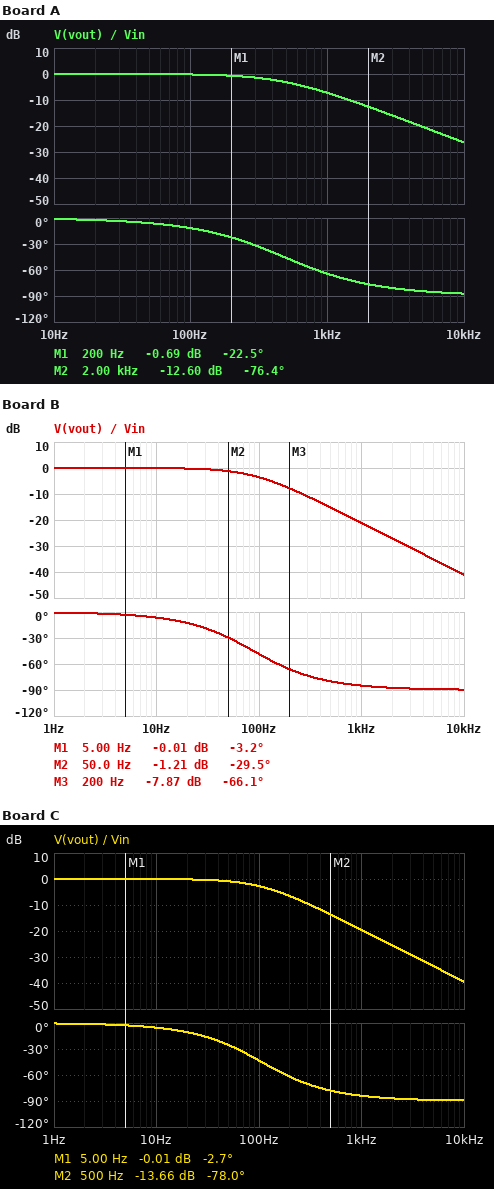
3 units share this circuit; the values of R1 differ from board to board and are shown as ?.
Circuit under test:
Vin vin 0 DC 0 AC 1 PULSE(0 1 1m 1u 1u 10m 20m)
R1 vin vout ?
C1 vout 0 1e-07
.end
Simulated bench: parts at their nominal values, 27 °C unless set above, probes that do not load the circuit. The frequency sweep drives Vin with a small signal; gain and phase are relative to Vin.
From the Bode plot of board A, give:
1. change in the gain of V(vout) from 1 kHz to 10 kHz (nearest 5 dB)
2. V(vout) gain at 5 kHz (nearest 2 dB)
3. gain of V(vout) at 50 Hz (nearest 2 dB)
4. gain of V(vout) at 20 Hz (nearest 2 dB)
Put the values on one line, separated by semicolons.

-20 dB; -20 dB; 0 dB; 0 dB
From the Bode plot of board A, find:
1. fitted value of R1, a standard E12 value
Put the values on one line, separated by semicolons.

3.3 kΩ
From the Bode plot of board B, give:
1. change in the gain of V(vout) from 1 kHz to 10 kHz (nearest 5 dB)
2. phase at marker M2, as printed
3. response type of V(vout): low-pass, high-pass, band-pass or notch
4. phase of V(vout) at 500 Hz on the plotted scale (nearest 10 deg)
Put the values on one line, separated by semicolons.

-20 dB; -29.5 deg; low-pass; -80 deg
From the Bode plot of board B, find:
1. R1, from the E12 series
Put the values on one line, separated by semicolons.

18 kΩ
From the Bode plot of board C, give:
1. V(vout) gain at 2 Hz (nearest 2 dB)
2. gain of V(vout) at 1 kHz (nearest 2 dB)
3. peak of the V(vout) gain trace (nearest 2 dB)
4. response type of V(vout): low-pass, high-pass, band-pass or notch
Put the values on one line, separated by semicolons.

0 dB; -20 dB; 0 dB; low-pass
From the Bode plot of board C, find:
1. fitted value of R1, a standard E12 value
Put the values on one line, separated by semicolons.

15 kΩ
